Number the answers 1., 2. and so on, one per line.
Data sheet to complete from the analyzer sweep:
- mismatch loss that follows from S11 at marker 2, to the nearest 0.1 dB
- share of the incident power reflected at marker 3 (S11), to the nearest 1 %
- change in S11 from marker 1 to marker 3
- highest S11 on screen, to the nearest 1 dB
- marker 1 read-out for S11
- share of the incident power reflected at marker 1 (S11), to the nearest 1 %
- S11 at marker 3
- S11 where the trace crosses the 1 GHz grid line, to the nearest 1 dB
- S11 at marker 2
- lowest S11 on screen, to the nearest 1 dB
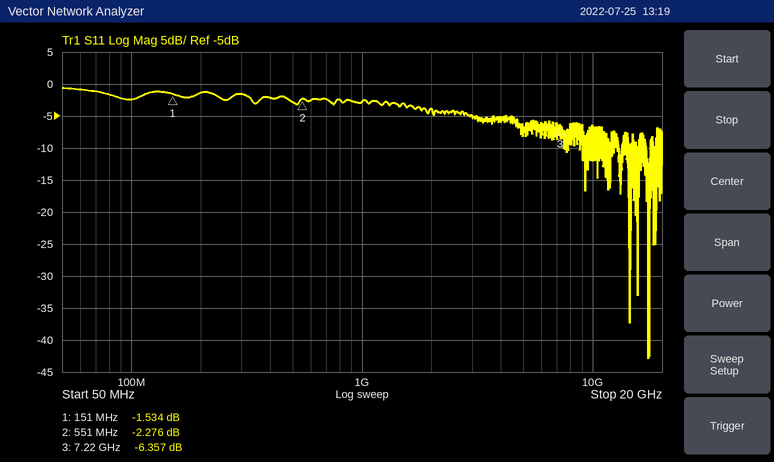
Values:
1. 3.9 dB
2. 23 %
3. -4.823 dB
4. -1 dB
5. -1.534 dB
6. 70 %
7. -6.357 dB
8. -3 dB
9. -2.276 dB
10. -43 dB
